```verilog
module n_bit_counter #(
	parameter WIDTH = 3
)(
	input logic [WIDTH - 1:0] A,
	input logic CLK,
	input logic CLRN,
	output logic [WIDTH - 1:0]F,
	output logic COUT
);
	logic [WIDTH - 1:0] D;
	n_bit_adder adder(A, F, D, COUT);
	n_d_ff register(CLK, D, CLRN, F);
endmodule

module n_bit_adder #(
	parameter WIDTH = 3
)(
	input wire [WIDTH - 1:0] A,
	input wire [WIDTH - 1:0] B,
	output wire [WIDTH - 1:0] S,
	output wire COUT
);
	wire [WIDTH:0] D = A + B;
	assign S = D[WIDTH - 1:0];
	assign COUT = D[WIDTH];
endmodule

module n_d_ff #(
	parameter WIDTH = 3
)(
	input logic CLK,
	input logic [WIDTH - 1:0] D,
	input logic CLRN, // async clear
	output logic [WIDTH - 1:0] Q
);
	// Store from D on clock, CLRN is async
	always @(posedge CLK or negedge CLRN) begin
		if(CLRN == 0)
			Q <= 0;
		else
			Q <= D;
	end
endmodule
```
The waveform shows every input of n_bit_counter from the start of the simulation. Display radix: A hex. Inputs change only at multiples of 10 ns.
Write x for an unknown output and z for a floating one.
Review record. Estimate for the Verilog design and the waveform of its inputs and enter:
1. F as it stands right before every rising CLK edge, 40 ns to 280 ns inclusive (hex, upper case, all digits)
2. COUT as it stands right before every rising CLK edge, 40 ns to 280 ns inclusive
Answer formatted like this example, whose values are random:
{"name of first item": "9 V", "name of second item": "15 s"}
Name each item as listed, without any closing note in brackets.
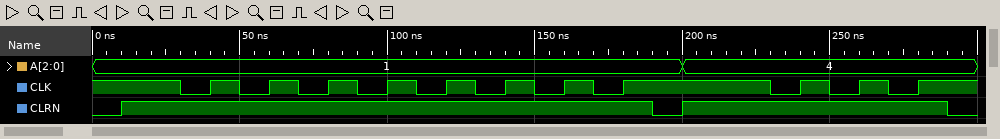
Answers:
{"F as it stands right before every rising CLK edge, 40 ns to 280 ns inclusive": "0, 1, 2, 3, 4, 5, 6, 7, 0, 4, 0", "COUT as it stands right before every rising CLK edge, 40 ns to 280 ns inclusive": "0 0 0 0 0 0 0 1 0 1 0"}
